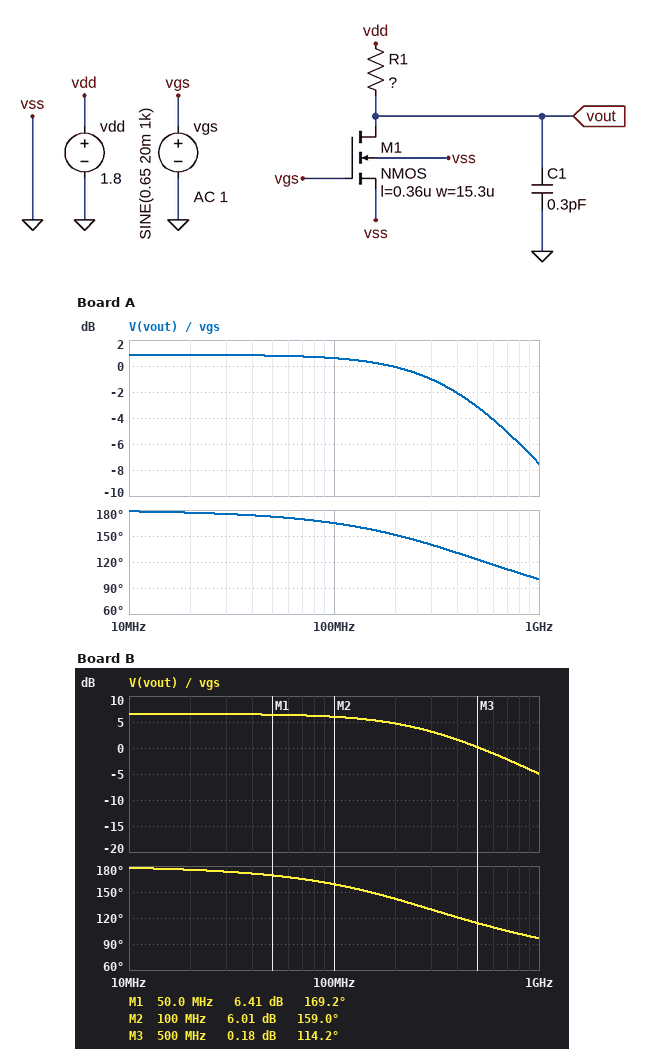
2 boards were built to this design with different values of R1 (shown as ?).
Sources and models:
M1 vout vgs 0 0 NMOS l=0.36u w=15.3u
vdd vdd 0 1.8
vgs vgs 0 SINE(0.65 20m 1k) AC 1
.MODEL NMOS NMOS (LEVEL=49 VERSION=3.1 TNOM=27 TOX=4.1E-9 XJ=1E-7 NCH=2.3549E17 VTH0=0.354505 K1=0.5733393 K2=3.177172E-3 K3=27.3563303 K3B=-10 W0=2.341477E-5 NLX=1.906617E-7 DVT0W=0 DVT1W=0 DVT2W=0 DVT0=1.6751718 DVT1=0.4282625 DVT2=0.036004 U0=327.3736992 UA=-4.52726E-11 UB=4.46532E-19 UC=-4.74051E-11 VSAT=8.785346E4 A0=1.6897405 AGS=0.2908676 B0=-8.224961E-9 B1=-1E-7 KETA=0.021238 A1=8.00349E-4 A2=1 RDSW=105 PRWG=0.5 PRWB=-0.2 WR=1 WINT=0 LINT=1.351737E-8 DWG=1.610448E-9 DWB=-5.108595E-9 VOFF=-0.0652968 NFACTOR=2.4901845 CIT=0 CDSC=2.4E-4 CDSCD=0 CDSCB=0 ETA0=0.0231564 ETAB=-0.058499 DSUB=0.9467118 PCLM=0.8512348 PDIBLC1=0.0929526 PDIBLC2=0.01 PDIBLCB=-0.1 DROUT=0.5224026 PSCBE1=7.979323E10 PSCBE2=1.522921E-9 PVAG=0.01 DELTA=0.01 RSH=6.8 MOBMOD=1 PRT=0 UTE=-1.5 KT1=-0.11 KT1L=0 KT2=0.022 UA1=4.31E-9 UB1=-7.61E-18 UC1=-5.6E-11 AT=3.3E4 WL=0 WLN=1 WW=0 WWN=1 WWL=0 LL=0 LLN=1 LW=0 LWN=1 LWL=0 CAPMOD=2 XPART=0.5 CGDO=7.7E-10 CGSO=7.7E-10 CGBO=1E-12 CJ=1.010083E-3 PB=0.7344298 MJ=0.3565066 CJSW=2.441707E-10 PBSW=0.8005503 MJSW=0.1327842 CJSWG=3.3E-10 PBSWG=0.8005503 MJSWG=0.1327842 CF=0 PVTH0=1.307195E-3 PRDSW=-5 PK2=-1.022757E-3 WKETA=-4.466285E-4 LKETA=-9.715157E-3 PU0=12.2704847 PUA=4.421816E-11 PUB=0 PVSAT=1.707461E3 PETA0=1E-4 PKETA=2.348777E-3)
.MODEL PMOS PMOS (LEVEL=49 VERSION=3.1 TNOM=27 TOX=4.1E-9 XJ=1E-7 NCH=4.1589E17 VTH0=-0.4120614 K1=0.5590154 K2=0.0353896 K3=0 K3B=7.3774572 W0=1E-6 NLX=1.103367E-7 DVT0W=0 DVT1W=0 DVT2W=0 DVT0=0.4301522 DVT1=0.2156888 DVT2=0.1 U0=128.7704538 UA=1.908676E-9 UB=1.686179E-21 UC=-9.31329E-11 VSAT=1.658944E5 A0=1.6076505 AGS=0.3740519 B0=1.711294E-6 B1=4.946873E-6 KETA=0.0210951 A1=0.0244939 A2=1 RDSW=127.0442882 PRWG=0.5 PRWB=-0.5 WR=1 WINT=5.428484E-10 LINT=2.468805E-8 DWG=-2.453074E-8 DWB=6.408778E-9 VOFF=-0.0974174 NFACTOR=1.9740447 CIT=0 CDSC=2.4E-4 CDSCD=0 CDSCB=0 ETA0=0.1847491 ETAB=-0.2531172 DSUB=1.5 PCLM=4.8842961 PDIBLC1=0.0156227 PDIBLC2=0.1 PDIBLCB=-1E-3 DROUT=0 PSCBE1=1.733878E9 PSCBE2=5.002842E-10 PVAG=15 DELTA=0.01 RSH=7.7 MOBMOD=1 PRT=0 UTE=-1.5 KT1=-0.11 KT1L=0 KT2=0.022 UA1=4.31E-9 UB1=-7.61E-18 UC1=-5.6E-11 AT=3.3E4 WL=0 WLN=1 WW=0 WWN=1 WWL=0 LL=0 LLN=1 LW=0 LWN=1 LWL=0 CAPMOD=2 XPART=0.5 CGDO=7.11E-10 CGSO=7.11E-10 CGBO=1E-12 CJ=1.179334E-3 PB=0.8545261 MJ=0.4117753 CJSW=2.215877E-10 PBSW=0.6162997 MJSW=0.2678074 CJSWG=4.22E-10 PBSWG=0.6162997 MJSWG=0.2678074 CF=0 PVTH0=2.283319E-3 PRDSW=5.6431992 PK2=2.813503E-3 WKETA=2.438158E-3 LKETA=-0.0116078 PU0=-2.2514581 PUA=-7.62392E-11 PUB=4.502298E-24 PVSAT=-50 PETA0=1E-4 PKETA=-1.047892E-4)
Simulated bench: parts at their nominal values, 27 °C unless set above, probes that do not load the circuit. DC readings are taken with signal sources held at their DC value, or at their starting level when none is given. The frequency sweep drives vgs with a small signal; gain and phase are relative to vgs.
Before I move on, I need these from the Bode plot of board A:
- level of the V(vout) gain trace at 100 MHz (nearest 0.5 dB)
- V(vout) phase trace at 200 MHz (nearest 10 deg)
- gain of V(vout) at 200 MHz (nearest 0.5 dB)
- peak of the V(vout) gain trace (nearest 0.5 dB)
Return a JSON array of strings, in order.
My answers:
["0.5 dB", "150 deg", "0 dB", "1.0 dB"]
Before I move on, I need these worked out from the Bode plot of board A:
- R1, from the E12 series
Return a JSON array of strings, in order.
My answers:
["18 kΩ"]
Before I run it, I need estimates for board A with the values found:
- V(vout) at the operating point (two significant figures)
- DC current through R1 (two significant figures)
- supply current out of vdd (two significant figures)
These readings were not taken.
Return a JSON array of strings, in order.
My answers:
["78 mV", "96 µA", "96 µA"]
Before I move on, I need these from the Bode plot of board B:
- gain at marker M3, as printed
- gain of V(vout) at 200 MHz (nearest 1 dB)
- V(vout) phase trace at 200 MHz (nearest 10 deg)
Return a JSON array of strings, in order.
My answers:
["0.18 dB", "5 dB", "140 deg"]
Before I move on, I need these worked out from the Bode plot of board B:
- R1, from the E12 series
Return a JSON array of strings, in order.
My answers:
["15 kΩ"]
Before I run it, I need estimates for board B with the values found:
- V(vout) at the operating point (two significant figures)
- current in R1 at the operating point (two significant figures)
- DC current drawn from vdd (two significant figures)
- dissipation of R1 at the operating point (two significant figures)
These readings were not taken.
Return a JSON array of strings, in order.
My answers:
["110 mV", "110 µA", "110 µA", "190 µW"]
